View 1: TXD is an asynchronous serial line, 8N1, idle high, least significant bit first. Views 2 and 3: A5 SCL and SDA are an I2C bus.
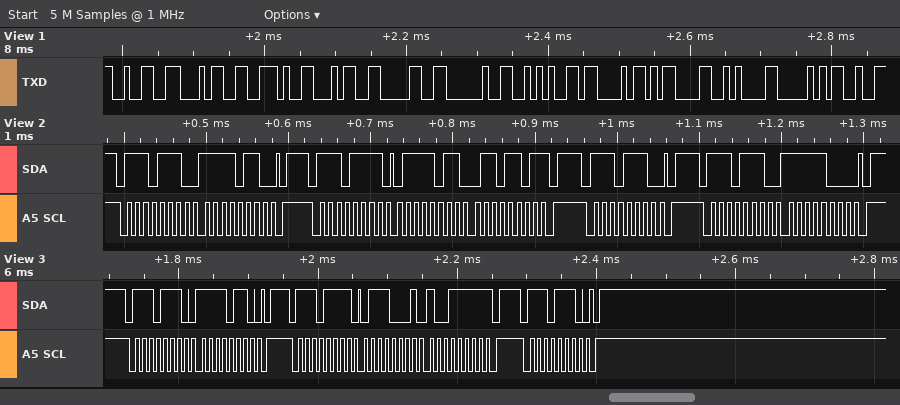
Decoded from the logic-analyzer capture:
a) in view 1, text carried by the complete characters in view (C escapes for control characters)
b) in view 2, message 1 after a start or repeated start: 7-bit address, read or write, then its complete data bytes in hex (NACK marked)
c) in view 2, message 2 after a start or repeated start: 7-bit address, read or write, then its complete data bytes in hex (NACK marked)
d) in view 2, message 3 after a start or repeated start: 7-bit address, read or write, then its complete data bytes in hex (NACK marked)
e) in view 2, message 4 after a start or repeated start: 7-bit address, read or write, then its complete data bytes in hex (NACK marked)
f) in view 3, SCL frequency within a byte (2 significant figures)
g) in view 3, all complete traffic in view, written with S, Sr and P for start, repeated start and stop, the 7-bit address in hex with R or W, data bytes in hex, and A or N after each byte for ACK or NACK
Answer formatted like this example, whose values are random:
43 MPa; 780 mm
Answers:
"24.40 *C\r\nP"; 0x77 write: F6; 0x77 read: 7B 6D NACK; 0x77 write; 0x77 write: F8; 100 kHz; S 77W A F6 A P S 77R A 71 A 9F N P S 77W A P
